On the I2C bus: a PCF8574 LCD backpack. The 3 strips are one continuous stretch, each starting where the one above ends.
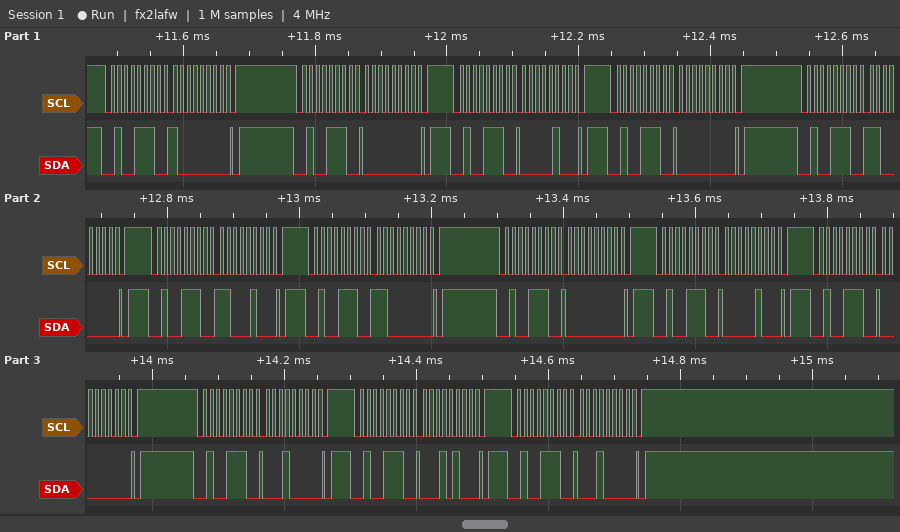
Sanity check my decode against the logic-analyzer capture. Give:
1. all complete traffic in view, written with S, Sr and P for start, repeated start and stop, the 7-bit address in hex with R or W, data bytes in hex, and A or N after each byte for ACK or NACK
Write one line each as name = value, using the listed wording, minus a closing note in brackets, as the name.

all complete traffic in view, written with S, Sr and P for start, repeated start and stop, the 7-bit address in hex with R or W, data bytes in hex, and A or N after each byte for ACK or NACK = S 27W A 80 A P S 27W A 00 A P S 27W A 04 A P S 27W A 00 A P S 27W A C0 A P S 27W A C4 A P S 27W A C0 A P S 27W A 00 A P S 27W A 04 A P S 27W A 00 A P S 27W A 10 A P S 27W A 14 A P S 27W A 10 A P
